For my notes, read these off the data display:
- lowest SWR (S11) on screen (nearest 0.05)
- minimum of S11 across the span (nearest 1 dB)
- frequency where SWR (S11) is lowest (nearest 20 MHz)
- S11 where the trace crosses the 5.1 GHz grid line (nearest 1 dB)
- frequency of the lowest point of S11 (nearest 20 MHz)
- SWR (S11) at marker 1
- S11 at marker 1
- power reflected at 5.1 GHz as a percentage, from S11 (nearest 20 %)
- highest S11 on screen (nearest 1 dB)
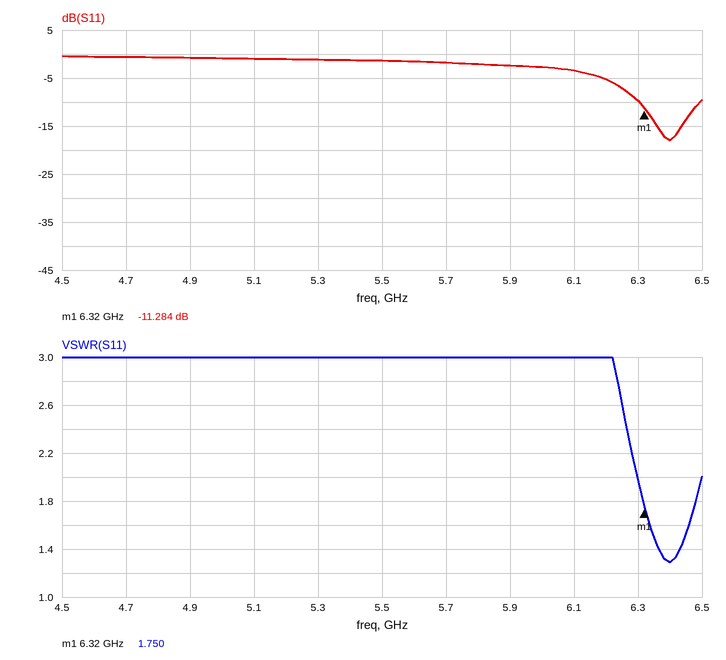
1.30
-18 dB
6.40 GHz
-1 dB
6.40 GHz
1.750
-11.284 dB
80 %
0 dB
